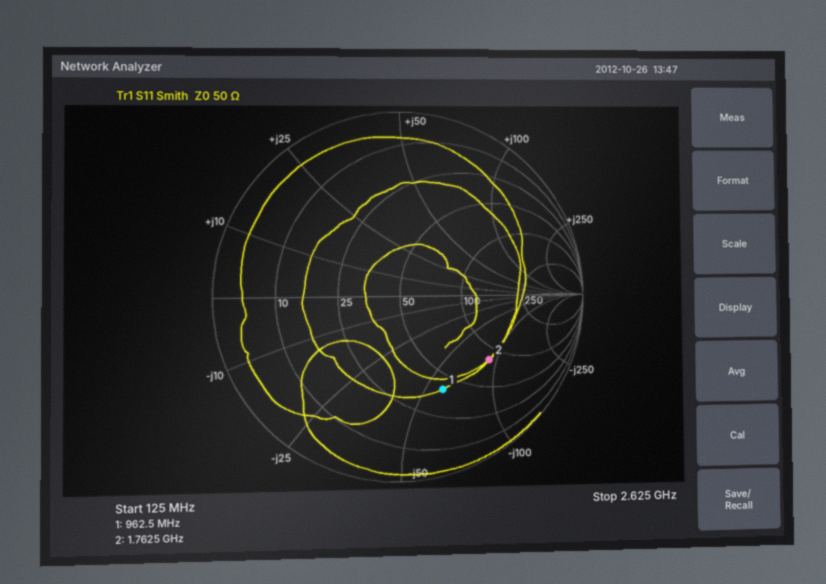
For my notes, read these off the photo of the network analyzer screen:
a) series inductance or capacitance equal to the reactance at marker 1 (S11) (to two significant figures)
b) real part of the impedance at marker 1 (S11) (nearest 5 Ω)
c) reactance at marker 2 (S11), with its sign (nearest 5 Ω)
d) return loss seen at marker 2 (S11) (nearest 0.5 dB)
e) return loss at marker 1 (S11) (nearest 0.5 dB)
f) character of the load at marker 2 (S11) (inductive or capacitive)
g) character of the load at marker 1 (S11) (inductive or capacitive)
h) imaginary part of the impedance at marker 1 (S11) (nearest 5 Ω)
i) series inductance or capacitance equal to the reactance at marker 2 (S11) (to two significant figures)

2.8 pF
40 Ω
-90 Ω
4.5 dB
5.0 dB
capacitive
capacitive
-60 Ω
1.0 pF
